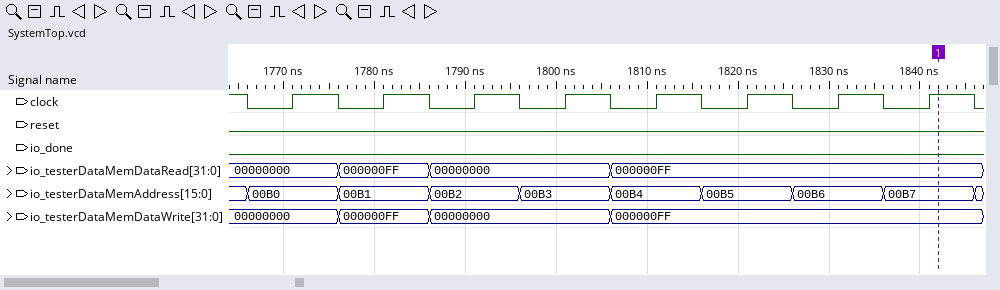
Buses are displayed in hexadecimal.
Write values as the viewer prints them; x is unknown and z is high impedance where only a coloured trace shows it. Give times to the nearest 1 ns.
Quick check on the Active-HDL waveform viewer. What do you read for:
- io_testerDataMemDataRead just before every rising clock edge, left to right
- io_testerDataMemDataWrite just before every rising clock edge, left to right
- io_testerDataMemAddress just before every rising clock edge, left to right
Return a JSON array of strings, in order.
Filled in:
["00000000, 000000FF, 00000000, 00000000, 000000FF, 000000FF, 000000FF, 000000FF", "00000000, 000000FF, 00000000, 00000000, 000000FF, 000000FF, 000000FF, 000000FF", "00B0, 00B1, 00B2, 00B3, 00B4, 00B5, 00B6, 00B7"]
